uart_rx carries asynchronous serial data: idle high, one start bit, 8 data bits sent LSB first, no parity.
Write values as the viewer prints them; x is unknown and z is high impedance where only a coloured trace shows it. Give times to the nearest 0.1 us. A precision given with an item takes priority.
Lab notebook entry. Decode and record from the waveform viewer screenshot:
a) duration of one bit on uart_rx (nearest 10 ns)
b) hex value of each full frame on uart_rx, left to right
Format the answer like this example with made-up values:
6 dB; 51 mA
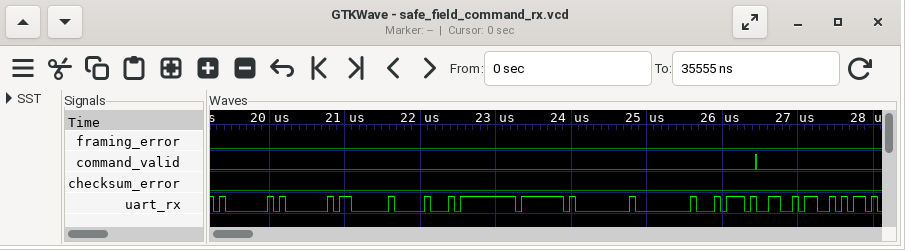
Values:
80 ns; 01, 01, 03, 10, FF, 7F, 00, 00, 74, A6, 6A
